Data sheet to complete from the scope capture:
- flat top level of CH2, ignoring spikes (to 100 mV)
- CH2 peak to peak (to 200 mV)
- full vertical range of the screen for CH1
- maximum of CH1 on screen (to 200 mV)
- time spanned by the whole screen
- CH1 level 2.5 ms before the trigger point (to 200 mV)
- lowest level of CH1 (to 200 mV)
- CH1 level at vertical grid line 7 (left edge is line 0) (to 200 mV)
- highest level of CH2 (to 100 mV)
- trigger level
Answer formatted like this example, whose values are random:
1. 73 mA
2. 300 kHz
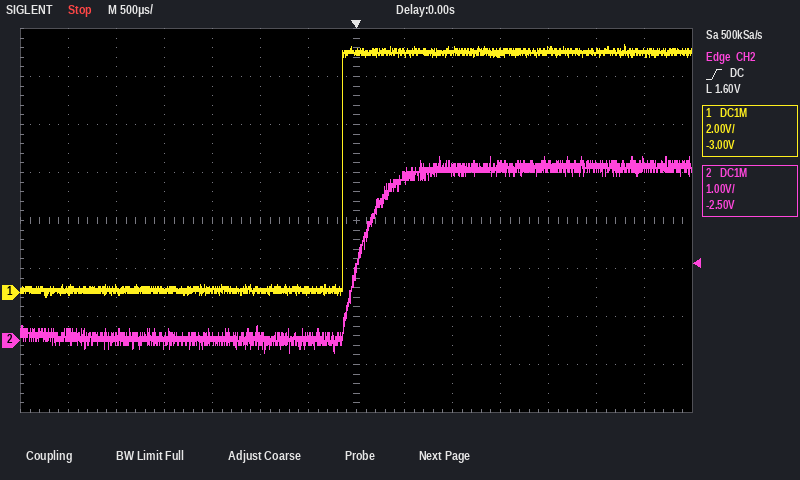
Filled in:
1. 3.6 V
2. 4.0 V
3. 16 V
4. 10.4 V
5. 7 ms
6. 200 mV
7. -200 mV
8. 10.0 V
9. 3.8 V
10. 1.60 V
